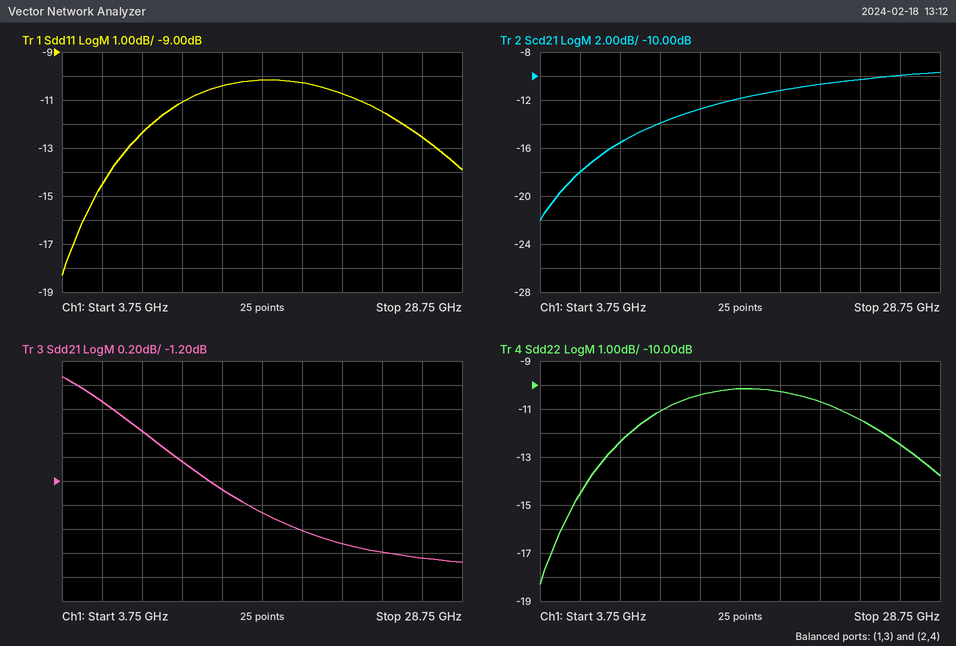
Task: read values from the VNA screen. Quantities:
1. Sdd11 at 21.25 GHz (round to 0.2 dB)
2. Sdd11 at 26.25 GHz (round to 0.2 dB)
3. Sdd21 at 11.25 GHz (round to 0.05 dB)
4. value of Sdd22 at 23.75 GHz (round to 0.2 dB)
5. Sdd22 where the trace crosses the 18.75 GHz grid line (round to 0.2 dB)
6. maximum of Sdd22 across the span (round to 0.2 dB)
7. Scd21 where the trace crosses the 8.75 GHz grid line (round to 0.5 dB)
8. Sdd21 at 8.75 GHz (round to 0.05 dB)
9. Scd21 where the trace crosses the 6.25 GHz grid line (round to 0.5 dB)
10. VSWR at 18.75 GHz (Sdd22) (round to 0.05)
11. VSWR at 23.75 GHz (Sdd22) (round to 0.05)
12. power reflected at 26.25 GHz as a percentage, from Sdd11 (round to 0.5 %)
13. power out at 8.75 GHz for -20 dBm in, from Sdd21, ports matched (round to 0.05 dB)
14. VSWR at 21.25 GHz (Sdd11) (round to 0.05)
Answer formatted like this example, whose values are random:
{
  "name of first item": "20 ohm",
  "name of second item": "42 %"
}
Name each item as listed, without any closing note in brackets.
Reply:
{
  "Sdd11 at 21.25 GHz": "-10.8 dB",
  "Sdd11 at 26.25 GHz": "-12.6 dB",
  "Sdd21 at 11.25 GHz": "-1.05 dB",
  "value of Sdd22 at 23.75 GHz": "-11.4 dB",
  "Sdd22 where the trace crosses the 18.75 GHz grid line": "-10.2 dB",
  "maximum of Sdd22 across the span": "-10.2 dB",
  "Scd21 where the trace crosses the 8.75 GHz grid line": "-15.5 dB",
  "Sdd21 at 8.75 GHz": "-0.80 dB",
  "Scd21 where the trace crosses the 6.25 GHz grid line": "-18.0 dB",
  "VSWR at 18.75 GHz (Sdd22)": "1.90",
  "VSWR at 23.75 GHz (Sdd22)": "1.75",
  "power reflected at 26.25 GHz as a percentage, from Sdd11": "5.5 %",
  "power out at 8.75 GHz for -20 dBm in, from Sdd21, ports matched": "-20.80 dBm",
  "VSWR at 21.25 GHz (Sdd11)": "1.80"
}
